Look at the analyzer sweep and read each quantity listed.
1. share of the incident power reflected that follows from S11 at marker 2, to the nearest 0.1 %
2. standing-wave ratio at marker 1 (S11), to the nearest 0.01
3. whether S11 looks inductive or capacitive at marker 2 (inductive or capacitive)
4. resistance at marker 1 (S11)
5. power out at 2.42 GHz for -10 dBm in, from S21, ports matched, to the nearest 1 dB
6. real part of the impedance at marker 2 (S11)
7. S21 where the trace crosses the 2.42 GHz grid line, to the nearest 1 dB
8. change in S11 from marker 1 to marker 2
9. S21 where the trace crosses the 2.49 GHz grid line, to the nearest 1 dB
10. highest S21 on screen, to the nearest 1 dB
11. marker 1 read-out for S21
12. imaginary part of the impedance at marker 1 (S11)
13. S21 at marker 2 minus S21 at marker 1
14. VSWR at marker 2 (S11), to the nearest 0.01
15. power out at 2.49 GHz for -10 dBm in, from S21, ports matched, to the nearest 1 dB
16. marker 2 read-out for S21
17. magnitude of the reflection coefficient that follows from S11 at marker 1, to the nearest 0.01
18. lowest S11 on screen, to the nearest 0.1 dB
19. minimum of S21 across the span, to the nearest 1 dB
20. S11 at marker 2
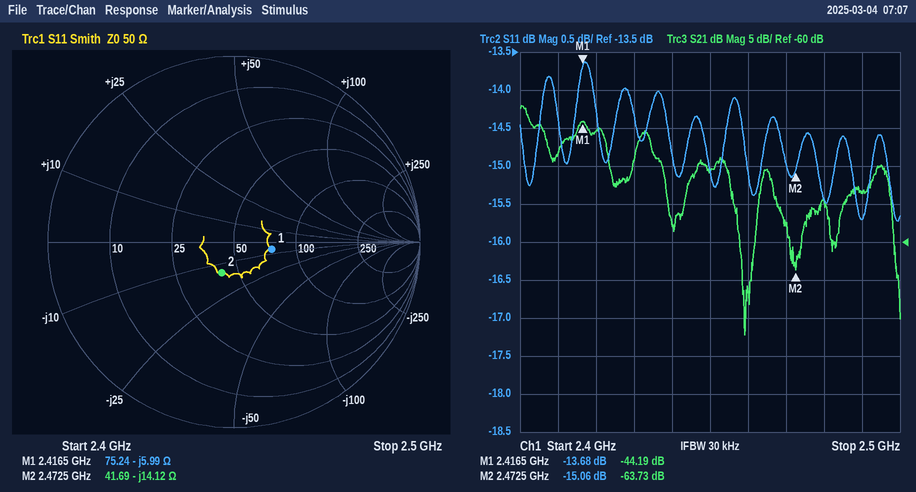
3.1 %
1.52
capacitive
75.24 Ω
-55 dBm
41.69 Ω
-45 dB
-1.38 dB
-53 dB
-42 dB
-44.19 dB
-5.99 Ω
-19.54 dB
1.43
-63 dBm
-63.73 dB
0.21
-15.7 dB
-72 dB
-15.06 dB
